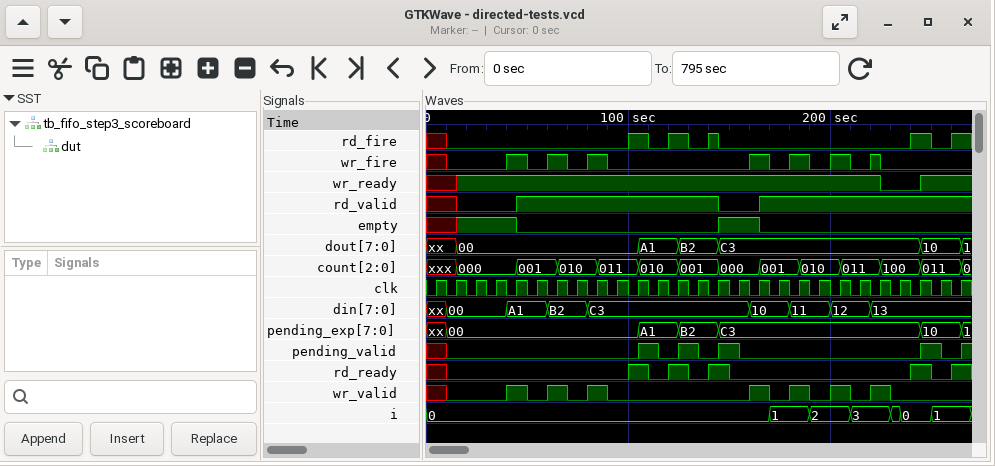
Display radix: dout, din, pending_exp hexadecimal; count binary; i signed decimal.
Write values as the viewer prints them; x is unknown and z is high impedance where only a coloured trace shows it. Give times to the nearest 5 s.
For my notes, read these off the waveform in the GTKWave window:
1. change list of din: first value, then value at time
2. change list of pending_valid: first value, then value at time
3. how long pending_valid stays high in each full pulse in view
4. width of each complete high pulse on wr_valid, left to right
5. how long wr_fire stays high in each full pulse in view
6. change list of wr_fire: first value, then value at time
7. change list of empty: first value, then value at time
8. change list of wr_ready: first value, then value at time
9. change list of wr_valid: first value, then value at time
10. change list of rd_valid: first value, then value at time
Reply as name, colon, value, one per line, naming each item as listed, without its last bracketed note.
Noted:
change list of din: first value, then value at time: xx, 00 at 10 s, A1 at 40 s, B2 at 60 s, C3 at 80 s, 10 at 160 s, 11 at 180 s, 12 at 200 s, 13 at 220 s
change list of pending_valid: first value, then value at time: x, 0 at 10 s, 1 at 105 s, 0 at 115 s, 1 at 125 s, 0 at 135 s, 1 at 145 s, 0 at 155 s, 1 at 245 s, 0 at 255 s, 1 at 265 s
how long pending_valid stays high in each full pulse in view: 10 s, 10 s, 10 s, 10 s
width of each complete high pulse on wr_valid, left to right: 10 s, 10 s, 10 s, 10 s, 10 s, 10 s, 10 s
how long wr_fire stays high in each full pulse in view: 10 s, 10 s, 10 s, 10 s, 10 s, 10 s, 5 s
change list of wr_fire: first value, then value at time: x, 0 at 10 s, 1 at 40 s, 0 at 50 s, 1 at 60 s, 0 at 70 s, 1 at 80 s, 0 at 90 s, 1 at 160 s, 0 at 170 s, 1 at 180 s, 0 at 190 s, 1 at 200 s, 0 at 210 s, 1 at 220 s, 0 at 225 s
change list of empty: first value, then value at time: x, 1 at 15 s, 0 at 45 s, 1 at 145 s, 0 at 165 s
change list of wr_ready: first value, then value at time: x, 1 at 15 s, 0 at 225 s, 1 at 245 s
change list of wr_valid: first value, then value at time: x, 0 at 10 s, 1 at 40 s, 0 at 50 s, 1 at 60 s, 0 at 70 s, 1 at 80 s, 0 at 90 s, 1 at 160 s, 0 at 170 s, 1 at 180 s, 0 at 190 s, 1 at 200 s, 0 at 210 s, 1 at 220 s, 0 at 230 s
change list of rd_valid: first value, then value at time: x, 0 at 15 s, 1 at 45 s, 0 at 145 s, 1 at 165 s
